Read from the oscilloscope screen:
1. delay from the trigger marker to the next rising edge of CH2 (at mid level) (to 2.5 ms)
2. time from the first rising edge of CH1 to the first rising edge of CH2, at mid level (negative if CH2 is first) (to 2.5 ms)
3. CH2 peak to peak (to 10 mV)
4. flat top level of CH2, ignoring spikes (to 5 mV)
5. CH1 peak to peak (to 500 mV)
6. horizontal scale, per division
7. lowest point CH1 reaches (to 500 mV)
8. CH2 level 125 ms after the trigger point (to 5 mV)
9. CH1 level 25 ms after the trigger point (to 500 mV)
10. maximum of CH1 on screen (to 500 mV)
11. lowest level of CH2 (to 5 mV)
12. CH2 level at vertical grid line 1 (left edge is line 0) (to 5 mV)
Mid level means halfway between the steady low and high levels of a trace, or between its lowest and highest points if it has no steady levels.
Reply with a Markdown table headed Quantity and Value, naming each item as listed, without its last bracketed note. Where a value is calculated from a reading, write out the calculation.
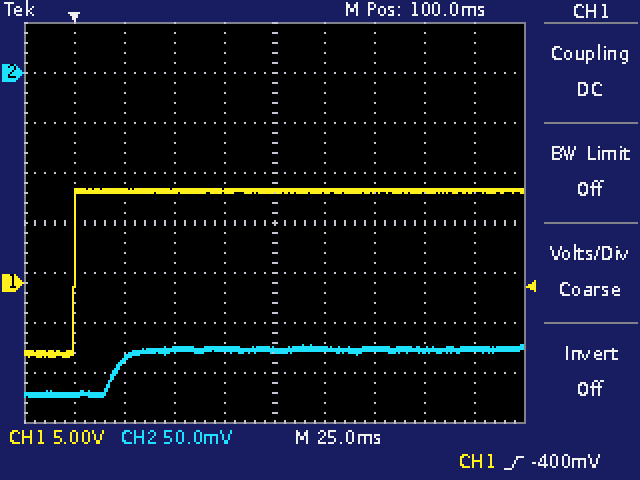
| Quantity | Value |
|---|---|
| delay from the trigger marker to the next rising edge of CH2 (at mid level) | 20.0 ms |
| time from the first rising edge of CH1 to the first rising edge of CH2, at mid level (negative if CH2 is first) | +20.0 ms |
| CH2 peak to peak | 50 mV |
| flat top level of CH2, ignoring spikes | -275 mV |
| CH1 peak to peak | 9.5 V − (-7.5 V) = 17.0 V |
| horizontal scale, per division | 25 ms |
| lowest point CH1 reaches | -7.5 V |
| CH2 level 125 ms after the trigger point | -275 mV |
| CH1 level 25 ms after the trigger point | 9.0 V |
| maximum of CH1 on screen | 9.5 V |
| lowest level of CH2 | -325 mV |
| CH2 level at vertical grid line 1 (left edge is line 0) | -320 mV |
